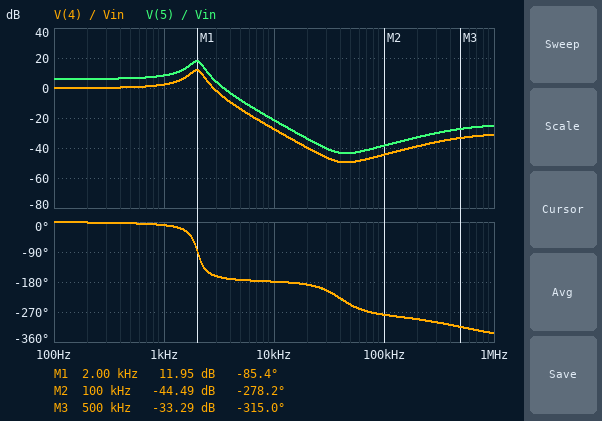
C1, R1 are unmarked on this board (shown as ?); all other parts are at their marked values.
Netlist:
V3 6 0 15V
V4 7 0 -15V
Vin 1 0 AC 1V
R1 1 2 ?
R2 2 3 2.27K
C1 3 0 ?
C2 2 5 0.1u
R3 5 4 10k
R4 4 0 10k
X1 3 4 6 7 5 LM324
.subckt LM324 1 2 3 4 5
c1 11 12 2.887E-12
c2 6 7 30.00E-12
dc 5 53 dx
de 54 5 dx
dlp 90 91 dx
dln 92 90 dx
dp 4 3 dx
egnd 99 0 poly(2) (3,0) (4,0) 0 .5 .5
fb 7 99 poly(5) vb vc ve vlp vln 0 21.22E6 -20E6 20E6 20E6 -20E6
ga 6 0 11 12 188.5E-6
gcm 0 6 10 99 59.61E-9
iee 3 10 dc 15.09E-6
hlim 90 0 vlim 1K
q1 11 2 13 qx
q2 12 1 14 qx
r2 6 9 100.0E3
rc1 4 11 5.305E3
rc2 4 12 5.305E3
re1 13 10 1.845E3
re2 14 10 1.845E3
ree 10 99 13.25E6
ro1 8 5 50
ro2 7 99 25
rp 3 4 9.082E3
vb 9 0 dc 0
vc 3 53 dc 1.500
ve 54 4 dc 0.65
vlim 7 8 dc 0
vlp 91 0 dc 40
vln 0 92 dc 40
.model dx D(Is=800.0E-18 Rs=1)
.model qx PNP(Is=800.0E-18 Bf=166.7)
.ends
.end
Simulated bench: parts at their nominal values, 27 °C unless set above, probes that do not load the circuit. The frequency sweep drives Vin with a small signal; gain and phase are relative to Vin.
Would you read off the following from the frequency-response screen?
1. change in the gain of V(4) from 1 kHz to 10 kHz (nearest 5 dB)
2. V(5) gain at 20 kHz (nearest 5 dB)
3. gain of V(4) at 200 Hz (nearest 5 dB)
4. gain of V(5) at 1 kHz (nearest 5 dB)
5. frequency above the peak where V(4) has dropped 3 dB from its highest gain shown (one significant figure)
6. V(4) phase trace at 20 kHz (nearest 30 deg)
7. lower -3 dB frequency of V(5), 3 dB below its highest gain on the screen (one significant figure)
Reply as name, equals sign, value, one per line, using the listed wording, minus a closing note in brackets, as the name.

change in the gain of V(4) from 1 kHz to 10 kHz = -30 dB
V(5) gain at 20 kHz = -35 dB
gain of V(4) at 200 Hz = 0 dB
gain of V(5) at 1 kHz = 10 dB
frequency above the peak where V(4) has dropped 3 dB from its highest gain shown = 2 kHz
V(4) phase trace at 20 kHz = -180 deg
lower -3 dB frequency of V(5), 3 dB below its highest gain on the screen = 2 kHz
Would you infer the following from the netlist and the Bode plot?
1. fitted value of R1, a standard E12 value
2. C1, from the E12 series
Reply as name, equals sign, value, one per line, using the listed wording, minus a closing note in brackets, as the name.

fitted value of R1, a standard E12 value = 820 Ω
C1, from the E12 series = 33 nF
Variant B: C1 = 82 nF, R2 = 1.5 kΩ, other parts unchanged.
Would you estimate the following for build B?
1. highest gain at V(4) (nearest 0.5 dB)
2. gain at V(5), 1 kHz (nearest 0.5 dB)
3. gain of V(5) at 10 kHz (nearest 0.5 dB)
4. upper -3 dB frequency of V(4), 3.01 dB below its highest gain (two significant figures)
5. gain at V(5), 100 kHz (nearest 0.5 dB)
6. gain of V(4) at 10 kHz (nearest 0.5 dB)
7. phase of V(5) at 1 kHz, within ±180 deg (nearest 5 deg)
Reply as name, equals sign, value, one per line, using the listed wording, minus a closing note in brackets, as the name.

highest gain at V(4) = 1.0 dB
gain at V(5), 1 kHz = 7.0 dB
gain of V(5) at 10 kHz = -26.0 dB
upper -3 dB frequency of V(4), 3.01 dB below its highest gain = 1.8 kHz
gain at V(5), 100 kHz = -38.5 dB
gain of V(4) at 10 kHz = -32.0 dB
phase of V(5) at 1 kHz, within ±180 deg = -50 deg
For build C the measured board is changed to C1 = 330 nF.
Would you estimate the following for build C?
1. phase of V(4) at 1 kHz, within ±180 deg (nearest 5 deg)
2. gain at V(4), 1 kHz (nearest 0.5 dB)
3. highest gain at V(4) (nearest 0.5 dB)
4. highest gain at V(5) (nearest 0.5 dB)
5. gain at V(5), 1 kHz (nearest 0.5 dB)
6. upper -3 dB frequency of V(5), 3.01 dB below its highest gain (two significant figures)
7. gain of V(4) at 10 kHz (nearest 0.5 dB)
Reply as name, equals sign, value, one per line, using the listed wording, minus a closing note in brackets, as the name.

phase of V(4) at 1 kHz, within ±180 deg = -105 deg
gain at V(4), 1 kHz = -15.5 dB
highest gain at V(4) = 0 dB
highest gain at V(5) = 6.0 dB
gain at V(5), 1 kHz = -9.5 dB
upper -3 dB frequency of V(5), 3.01 dB below its highest gain = 180 Hz
gain of V(4) at 10 kHz = -48.0 dB
